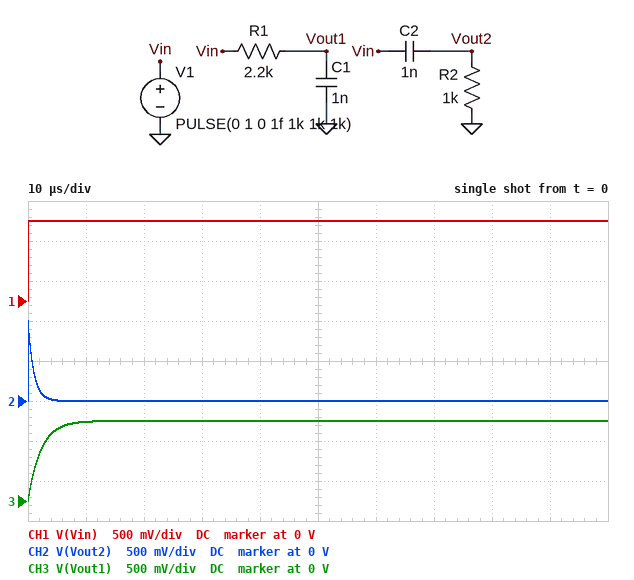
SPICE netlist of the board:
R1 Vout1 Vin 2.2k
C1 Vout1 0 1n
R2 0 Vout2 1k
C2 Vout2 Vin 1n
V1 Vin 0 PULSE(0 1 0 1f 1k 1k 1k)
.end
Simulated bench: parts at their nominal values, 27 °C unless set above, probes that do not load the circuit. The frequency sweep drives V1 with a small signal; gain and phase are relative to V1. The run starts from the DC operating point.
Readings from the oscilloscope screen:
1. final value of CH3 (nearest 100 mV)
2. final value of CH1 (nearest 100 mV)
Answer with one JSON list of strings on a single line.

["1.0 V", "1.0 V"]
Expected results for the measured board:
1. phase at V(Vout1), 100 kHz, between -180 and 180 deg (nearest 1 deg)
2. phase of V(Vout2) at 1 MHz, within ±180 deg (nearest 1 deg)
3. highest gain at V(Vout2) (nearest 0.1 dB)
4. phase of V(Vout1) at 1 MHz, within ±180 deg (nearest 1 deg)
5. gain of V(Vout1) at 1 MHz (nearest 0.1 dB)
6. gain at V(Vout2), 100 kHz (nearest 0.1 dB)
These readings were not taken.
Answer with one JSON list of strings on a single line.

["-54 deg", "9 deg", "0 dB", "-86 deg", "-22.8 dB", "-5.5 dB"]
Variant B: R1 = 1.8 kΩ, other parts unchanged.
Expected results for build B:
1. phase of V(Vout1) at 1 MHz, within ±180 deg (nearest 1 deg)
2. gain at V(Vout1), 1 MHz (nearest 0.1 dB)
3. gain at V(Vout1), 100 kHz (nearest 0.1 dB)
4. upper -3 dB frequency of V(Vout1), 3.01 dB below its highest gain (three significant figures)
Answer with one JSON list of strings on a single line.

["-85 deg", "-21.1 dB", "-3.6 dB", "88.4 kHz"]
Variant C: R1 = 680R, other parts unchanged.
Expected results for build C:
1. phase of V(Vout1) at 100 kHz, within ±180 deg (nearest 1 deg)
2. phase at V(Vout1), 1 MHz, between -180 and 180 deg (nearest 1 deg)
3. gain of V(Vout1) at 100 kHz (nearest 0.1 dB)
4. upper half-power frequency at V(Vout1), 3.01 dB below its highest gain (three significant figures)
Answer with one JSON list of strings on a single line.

["-23 deg", "-77 deg", "-0.7 dB", "234 kHz"]
